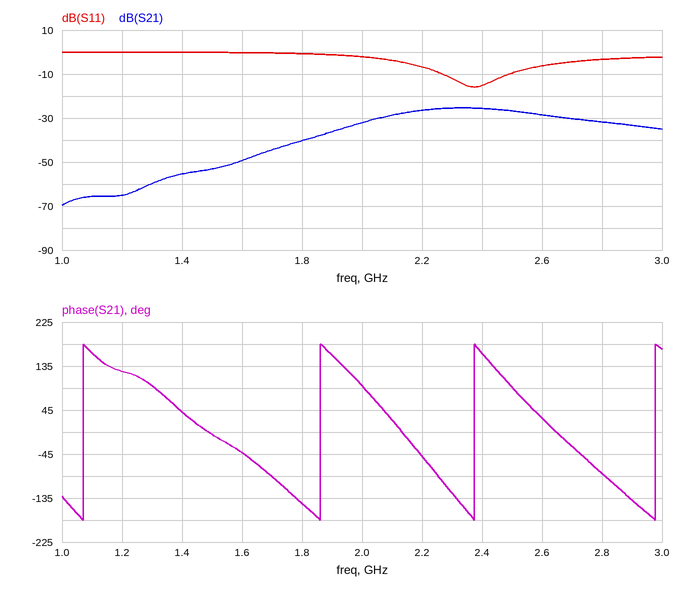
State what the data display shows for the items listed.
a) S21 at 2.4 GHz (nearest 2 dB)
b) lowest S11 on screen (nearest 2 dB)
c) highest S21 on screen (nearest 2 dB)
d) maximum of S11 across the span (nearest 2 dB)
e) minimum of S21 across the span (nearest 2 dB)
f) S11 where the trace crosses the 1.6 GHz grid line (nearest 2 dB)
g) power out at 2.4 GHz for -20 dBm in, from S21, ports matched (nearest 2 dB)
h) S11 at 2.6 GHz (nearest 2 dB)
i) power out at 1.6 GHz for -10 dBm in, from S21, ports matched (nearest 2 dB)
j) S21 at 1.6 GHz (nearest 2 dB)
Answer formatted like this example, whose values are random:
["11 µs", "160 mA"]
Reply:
["-26 dB", "-16 dB", "-26 dB", "0 dB", "-70 dB", "0 dB", "-46 dBm", "-6 dB", "-60 dBm", "-50 dB"]
